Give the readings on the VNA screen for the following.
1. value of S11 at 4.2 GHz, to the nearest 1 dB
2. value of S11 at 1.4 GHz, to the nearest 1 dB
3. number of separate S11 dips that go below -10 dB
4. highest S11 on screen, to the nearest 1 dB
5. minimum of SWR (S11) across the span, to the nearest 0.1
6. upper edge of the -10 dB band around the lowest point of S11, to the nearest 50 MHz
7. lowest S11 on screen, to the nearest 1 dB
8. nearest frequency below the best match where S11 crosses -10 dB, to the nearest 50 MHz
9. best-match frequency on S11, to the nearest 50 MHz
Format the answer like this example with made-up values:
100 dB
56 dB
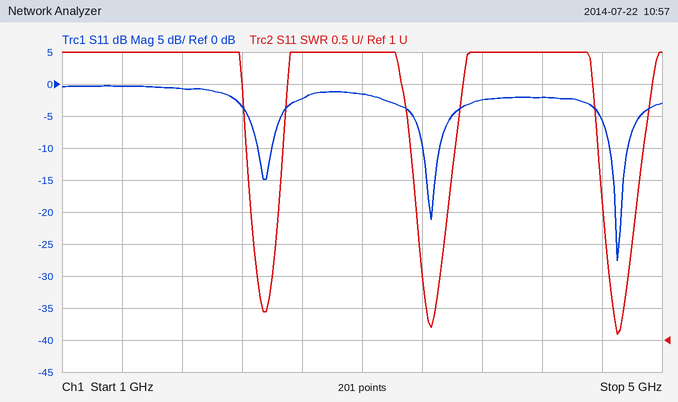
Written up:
-2 dB
0 dB
3
0 dB
1.1
4.75 GHz
-28 dB
4.65 GHz
4.70 GHz
